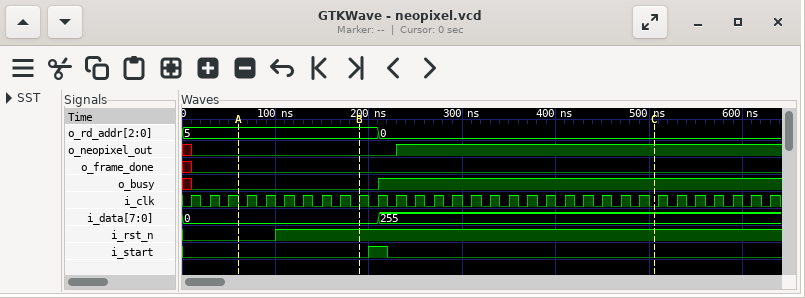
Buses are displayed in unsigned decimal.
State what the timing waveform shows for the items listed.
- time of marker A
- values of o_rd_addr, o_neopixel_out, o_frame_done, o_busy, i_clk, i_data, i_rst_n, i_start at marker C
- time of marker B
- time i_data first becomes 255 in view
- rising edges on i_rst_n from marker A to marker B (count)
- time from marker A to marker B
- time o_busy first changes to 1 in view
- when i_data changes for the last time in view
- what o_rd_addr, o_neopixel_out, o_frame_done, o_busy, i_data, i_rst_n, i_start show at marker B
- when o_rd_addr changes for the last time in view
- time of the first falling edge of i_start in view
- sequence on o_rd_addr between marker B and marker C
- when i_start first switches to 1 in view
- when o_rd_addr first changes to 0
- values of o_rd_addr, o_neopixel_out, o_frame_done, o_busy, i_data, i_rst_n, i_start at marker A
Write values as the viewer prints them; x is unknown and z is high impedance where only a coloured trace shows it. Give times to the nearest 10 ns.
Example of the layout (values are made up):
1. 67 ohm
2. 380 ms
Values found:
1. 60 ns
2. o_rd_addr=0, o_neopixel_out=1, o_frame_done=0, o_busy=1, i_clk=0, i_data=255, i_rst_n=1, i_start=0
3. 190 ns
4. 210 ns
5. 1
6. 130 ns
7. 210 ns
8. 210 ns
9. o_rd_addr=5, o_neopixel_out=0, o_frame_done=0, o_busy=0, i_data=0, i_rst_n=1, i_start=0
10. 210 ns
11. 220 ns
12. 5, 0
13. 200 ns
14. 210 ns
15. o_rd_addr=5, o_neopixel_out=0, o_frame_done=0, o_busy=0, i_data=0, i_rst_n=0, i_start=0
